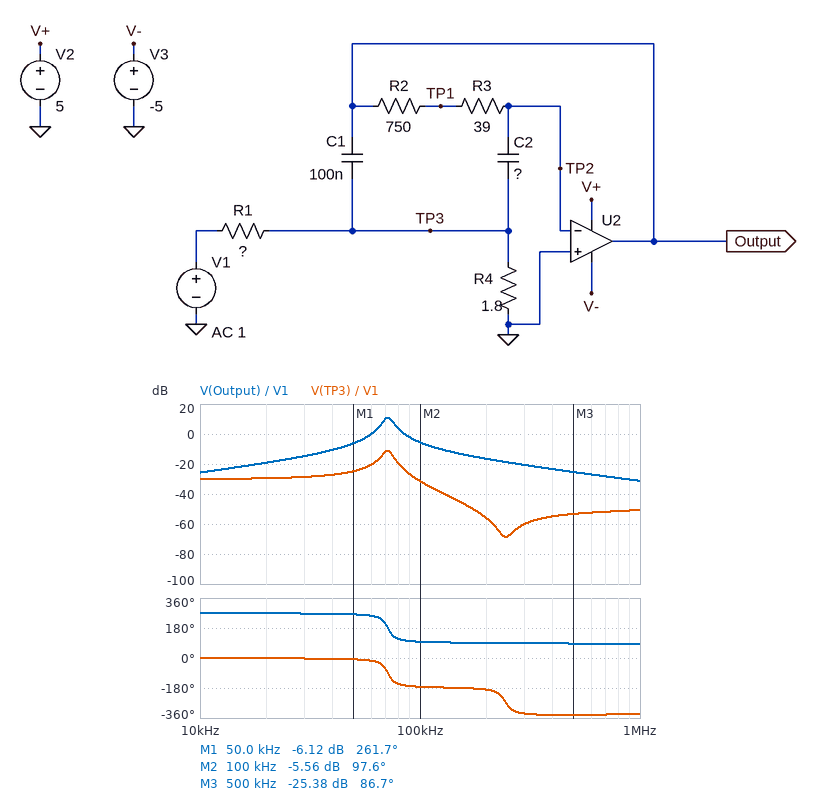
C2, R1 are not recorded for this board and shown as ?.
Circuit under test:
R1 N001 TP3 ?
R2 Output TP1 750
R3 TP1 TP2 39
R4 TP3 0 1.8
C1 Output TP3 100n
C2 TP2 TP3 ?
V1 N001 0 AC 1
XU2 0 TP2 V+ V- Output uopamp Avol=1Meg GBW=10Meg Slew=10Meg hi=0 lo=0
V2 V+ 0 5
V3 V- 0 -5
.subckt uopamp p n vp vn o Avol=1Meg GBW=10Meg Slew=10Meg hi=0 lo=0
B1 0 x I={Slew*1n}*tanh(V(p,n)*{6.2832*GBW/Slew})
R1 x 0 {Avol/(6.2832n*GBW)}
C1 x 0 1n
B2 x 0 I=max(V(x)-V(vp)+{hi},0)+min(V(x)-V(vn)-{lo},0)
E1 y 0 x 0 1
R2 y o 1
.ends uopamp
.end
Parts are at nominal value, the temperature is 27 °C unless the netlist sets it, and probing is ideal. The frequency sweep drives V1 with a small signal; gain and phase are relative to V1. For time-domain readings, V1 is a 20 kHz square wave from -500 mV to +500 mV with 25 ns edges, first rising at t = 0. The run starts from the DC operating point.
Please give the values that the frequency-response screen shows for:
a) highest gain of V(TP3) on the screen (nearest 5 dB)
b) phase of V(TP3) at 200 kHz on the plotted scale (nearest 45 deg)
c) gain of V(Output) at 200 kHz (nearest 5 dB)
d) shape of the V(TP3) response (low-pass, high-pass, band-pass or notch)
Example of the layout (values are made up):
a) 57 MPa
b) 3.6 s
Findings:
a) -10 dB
b) -180 deg
c) -15 dB
d) band-pass
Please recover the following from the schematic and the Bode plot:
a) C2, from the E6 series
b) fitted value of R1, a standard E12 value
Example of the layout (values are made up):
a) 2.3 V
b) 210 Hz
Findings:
a) 33 nF
b) 56 Ω
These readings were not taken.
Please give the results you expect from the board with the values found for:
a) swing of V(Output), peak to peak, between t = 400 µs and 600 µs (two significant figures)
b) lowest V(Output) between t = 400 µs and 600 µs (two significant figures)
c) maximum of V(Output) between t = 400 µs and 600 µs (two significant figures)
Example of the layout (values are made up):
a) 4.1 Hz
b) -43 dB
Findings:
a) 550 mV
b) -280 mV
c) 280 mV
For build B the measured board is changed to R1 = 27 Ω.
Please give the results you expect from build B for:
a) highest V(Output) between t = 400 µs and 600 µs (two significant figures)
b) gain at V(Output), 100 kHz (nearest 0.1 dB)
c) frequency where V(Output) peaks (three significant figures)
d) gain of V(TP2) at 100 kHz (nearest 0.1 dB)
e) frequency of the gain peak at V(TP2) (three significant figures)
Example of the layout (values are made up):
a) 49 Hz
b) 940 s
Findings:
a) 530 mV
b) 1.0 dB
c) 72.6 kHz
d) -38.9 dB
e) 72.8 kHz
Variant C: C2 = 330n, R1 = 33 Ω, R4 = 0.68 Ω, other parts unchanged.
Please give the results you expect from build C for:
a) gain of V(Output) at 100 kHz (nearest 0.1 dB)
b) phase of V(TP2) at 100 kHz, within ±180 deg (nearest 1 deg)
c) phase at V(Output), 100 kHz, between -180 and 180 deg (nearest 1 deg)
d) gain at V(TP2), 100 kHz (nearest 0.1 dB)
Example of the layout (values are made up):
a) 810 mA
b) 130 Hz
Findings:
a) -7.1 dB
b) 4 deg
c) 90 deg
d) -47.1 dB
